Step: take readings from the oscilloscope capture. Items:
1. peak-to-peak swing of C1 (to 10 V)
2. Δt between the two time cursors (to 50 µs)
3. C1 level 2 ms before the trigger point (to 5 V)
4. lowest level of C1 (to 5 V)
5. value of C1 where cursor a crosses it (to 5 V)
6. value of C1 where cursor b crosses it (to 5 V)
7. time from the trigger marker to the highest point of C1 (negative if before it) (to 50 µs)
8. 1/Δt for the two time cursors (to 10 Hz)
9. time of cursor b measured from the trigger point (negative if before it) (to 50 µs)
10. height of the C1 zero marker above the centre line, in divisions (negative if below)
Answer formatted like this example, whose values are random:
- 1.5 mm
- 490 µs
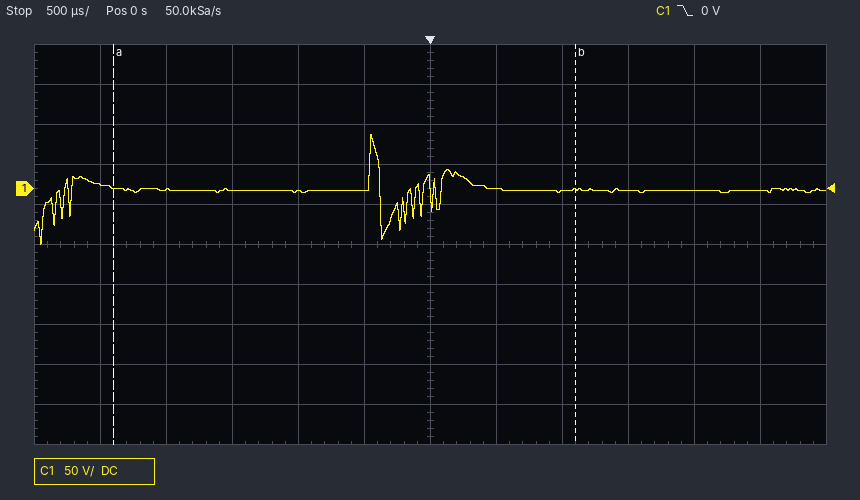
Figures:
- 140 V
- 3.50 ms
- 0 V
- -70 V
- 0 V
- 0 V
- -450 µs
- 290 Hz
- +1.10 ms
- +1.4 div
